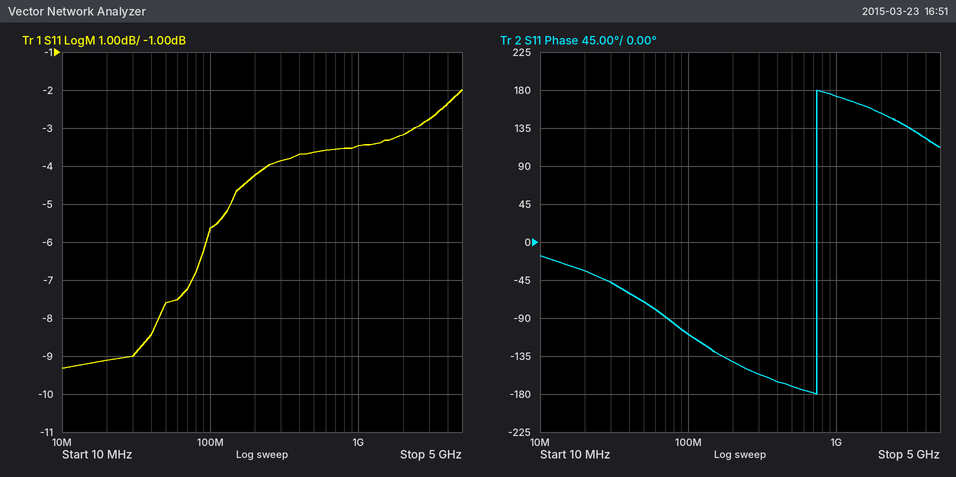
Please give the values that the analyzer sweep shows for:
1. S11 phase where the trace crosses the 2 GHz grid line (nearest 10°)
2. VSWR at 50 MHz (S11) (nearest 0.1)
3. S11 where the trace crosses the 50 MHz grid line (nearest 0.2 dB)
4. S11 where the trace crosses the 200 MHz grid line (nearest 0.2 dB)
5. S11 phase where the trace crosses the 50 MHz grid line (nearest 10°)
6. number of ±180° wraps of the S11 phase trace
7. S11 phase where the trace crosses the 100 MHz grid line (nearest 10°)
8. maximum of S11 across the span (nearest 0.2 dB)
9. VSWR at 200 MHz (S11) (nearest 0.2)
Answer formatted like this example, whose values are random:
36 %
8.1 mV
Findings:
150°
2.4
-7.6 dB
-4.2 dB
-70°
1
-110°
-2.0 dB
4.2
